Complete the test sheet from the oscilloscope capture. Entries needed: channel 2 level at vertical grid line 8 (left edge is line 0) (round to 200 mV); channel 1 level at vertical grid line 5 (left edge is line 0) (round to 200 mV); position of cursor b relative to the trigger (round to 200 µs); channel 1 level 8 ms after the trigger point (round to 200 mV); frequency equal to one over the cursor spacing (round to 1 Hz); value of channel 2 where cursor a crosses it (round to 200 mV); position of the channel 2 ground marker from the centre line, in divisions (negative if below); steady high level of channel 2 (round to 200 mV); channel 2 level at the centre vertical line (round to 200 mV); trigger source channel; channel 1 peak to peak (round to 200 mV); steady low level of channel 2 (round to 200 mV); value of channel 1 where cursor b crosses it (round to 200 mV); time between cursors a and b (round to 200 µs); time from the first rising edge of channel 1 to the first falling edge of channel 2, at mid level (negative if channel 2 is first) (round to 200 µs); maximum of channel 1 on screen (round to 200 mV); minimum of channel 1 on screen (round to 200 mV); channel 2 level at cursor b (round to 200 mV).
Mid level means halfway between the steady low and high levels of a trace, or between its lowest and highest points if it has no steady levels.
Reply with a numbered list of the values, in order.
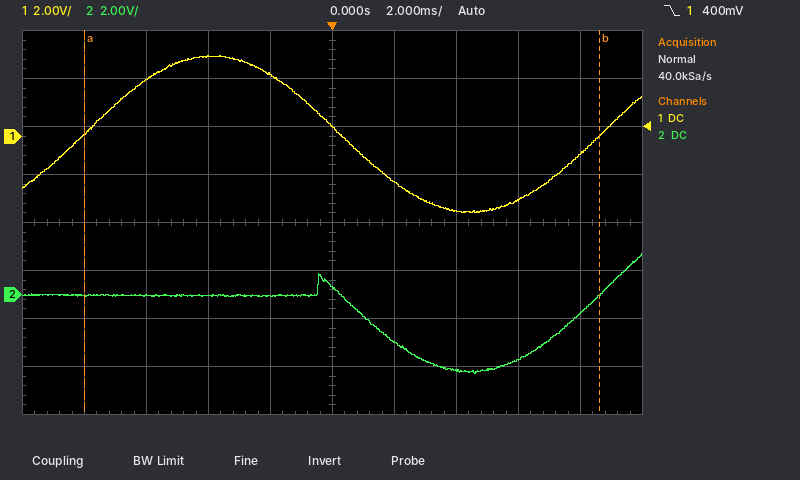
1. -2.8 V
2. 400 mV
3. +8.6 ms
4. -800 mV
5. 60 Hz
6. 0.0 V
7. -1.5 div
8. 0.0 V
9. 400 mV
10. channel 1
11. 6.6 V
12. -3.2 V
13. 0.0 V
14. 16.6 ms
15. +9.6 ms
16. 3.4 V
17. -3.2 V
18. 0.0 V
